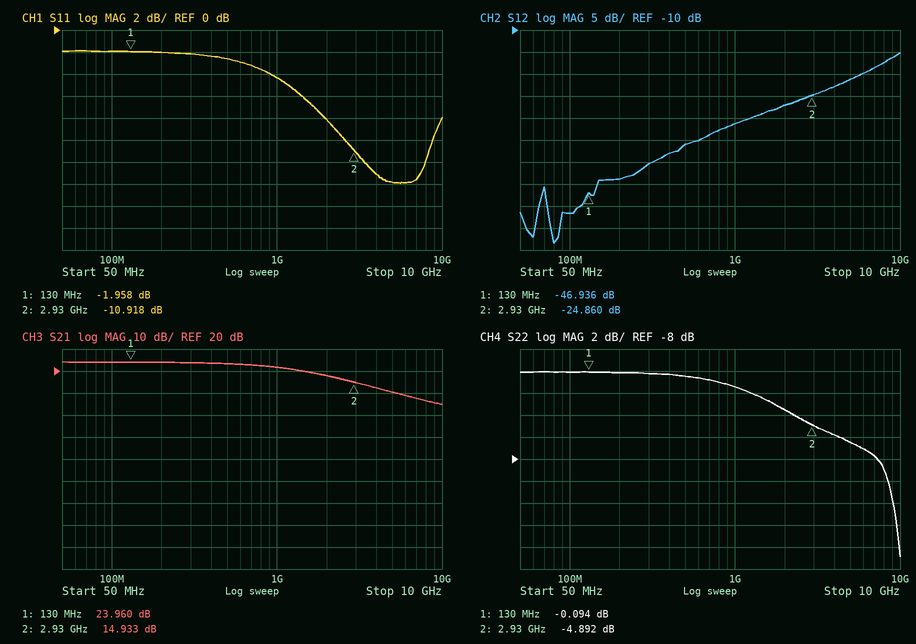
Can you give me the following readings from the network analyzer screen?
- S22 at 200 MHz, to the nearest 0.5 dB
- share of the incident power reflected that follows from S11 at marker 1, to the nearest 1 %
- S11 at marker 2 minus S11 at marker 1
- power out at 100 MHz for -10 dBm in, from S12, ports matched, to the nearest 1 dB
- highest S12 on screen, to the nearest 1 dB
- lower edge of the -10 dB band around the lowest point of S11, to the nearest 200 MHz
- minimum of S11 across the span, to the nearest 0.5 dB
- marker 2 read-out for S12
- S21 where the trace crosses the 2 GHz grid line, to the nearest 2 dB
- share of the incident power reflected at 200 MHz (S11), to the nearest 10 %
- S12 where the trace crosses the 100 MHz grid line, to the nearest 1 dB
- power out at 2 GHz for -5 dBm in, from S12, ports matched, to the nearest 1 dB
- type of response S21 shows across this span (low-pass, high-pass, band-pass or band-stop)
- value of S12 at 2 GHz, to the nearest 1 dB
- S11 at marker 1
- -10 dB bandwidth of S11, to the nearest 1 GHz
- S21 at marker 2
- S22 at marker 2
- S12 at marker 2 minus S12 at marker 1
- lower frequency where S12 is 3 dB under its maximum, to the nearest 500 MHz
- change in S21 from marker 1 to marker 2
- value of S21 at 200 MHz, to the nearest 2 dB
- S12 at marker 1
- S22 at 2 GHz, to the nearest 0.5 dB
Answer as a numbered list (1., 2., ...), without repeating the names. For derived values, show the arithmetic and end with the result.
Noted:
1. 0.0 dB
2. 10^(-1.958/10) ≈ 64 %
3. -10.918 − (-1.958) = -8.960 dB
4. -10 dBm + (-52 dB) = -62 dBm
5. -15 dB
6. 2.6 GHz
7. -14.0 dB
8. -24.860 dB
9. 18 dB
10. 10^(-2/10) ≈ 63.1 %, so 60 % to the nearest 10 %
11. -52 dB
12. -5 dBm + (-27 dB) = -32 dBm
13. low-pass
14. -27 dB
15. -1.958 dB
16. 9 GHz − 2.6 GHz = 6.4 GHz
17. 14.933 dB
18. -4.892 dB
19. -24.86 − (-46.936) = 22.076 dB
20. 7.5 GHz
21. 14.933 − (23.96) = -9.027 dB
22. 24 dB
23. -46.936 dB
24. -3.5 dB
